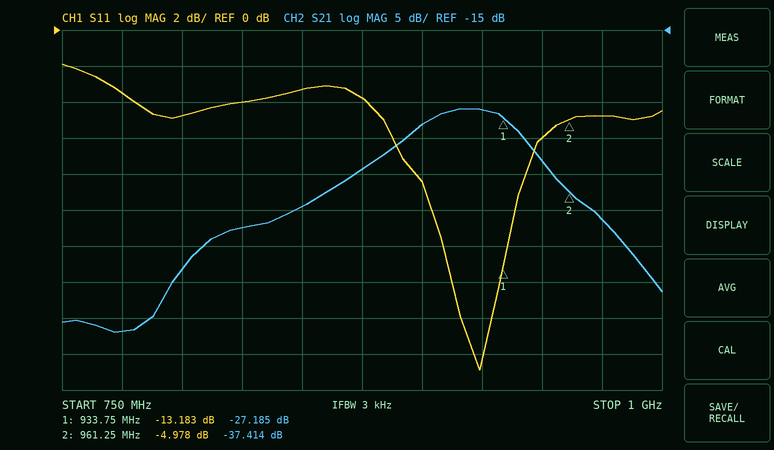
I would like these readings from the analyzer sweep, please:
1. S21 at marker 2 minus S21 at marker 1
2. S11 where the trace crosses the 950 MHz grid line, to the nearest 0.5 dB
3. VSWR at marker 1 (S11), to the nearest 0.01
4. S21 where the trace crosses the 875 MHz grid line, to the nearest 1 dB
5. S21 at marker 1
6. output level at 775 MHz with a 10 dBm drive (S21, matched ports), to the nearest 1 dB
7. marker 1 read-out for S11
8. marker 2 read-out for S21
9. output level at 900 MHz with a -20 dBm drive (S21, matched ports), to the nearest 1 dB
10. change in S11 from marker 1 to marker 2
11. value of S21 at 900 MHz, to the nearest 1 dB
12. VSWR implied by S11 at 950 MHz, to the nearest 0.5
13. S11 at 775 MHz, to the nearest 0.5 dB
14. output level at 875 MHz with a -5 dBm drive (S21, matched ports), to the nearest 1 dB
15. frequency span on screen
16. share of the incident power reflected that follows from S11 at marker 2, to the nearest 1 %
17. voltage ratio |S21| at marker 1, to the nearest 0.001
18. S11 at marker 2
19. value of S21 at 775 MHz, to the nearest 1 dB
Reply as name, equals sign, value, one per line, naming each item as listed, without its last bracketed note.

S21 at marker 2 minus S21 at marker 1 = -10.229 dB
S11 where the trace crosses the 950 MHz grid line, to the nearest 0.5 dB = -6.0 dB
VSWR at marker 1 (S11), to the nearest 0.01 = 1.56
S21 where the trace crosses the 875 MHz grid line, to the nearest 1 dB = -34 dB
S21 at marker 1 = -27.185 dB
output level at 775 MHz with a 10 dBm drive (S21, matched ports), to the nearest 1 dB = -47 dBm
marker 1 read-out for S11 = -13.183 dB
marker 2 read-out for S21 = -37.414 dB
output level at 900 MHz with a -20 dBm drive (S21, matched ports), to the nearest 1 dB = -48 dBm
change in S11 from marker 1 to marker 2 = 8.205 dB
value of S21 at 900 MHz, to the nearest 1 dB = -28 dB
VSWR implied by S11 at 950 MHz, to the nearest 0.5 = 3.0
S11 at 775 MHz, to the nearest 0.5 dB = -3.5 dB
output level at 875 MHz with a -5 dBm drive (S21, matched ports), to the nearest 1 dB = -39 dBm
frequency span on screen = 250 MHz
share of the incident power reflected that follows from S11 at marker 2, to the nearest 1 % = 32 %
voltage ratio |S21| at marker 1, to the nearest 0.001 = 0.044
S11 at marker 2 = -4.978 dB
value of S21 at 775 MHz, to the nearest 1 dB = -57 dB
